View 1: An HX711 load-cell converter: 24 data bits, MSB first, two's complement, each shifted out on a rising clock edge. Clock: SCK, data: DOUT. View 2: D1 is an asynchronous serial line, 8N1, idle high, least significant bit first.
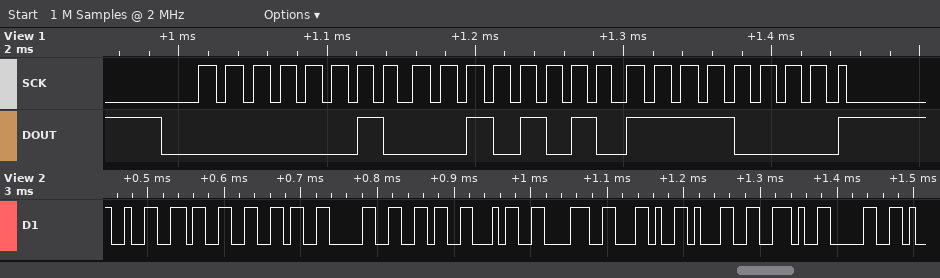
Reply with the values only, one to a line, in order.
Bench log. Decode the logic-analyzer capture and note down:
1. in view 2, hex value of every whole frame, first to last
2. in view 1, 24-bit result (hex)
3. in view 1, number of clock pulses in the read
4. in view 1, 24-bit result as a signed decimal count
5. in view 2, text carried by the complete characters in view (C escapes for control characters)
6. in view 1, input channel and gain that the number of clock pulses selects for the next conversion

32 33 36 30 36 34 38 2C 31 2E 30
0x022AF0
25
142064
"2360648,1.0"
channel A, gain 128
